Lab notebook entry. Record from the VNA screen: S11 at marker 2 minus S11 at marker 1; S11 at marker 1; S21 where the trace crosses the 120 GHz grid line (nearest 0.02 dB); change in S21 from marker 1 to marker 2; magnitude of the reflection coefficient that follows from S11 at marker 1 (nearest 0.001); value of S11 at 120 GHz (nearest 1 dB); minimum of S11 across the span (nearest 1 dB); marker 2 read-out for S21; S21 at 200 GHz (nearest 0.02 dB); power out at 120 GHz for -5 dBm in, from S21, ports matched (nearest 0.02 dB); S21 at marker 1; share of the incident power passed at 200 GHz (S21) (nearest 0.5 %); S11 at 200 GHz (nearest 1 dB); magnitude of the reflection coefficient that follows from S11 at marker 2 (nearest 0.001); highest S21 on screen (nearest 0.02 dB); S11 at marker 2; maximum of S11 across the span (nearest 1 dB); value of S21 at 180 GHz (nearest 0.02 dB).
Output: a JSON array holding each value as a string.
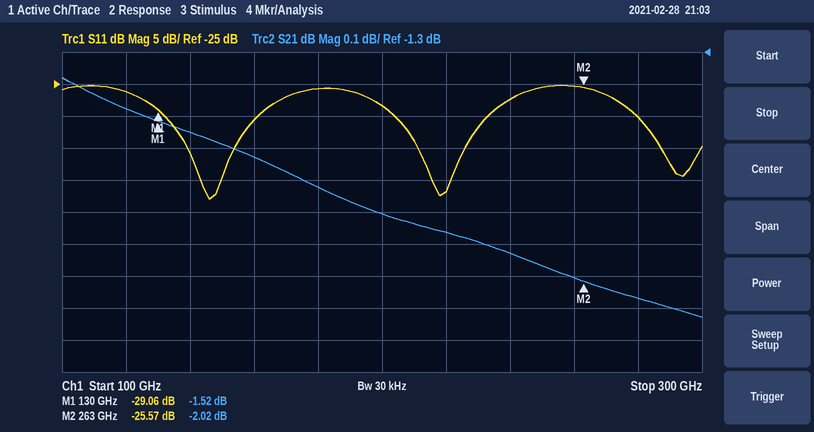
["3.49 dB", "-29.06 dB", "-1.48 dB", "-0.50 dB", "0.035", "-26 dB", "-43 dB", "-2.02 dB", "-1.80 dB", "-6.48 dBm", "-1.52 dB", "66.0 %", "-28 dB", "0.053", "-1.38 dB", "-25.57 dB", "-25 dB", "-1.72 dB"]
